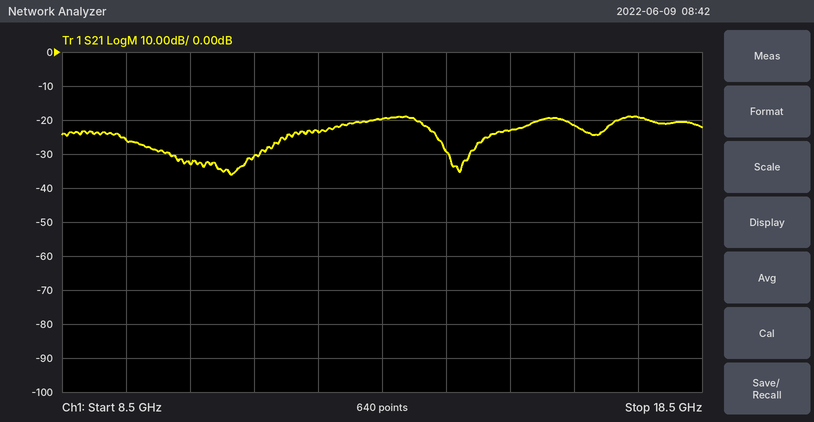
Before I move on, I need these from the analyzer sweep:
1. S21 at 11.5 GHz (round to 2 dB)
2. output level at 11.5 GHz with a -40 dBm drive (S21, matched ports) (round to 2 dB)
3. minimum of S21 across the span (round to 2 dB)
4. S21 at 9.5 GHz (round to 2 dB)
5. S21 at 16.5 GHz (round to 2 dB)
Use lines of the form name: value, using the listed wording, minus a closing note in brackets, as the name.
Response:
S21 at 11.5 GHz: -30 dB
output level at 11.5 GHz with a -40 dBm drive (S21, matched ports): -70 dBm
minimum of S21 across the span: -36 dB
S21 at 9.5 GHz: -26 dB
S21 at 16.5 GHz: -22 dB
